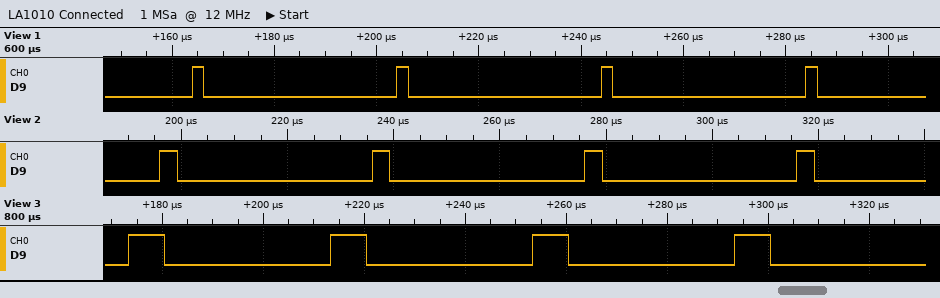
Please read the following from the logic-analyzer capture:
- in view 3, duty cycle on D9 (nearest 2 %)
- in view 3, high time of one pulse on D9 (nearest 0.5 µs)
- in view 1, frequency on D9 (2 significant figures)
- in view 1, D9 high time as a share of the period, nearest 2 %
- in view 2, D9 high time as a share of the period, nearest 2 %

18 %
7.0 µs
25 kHz
6 %
8 %
